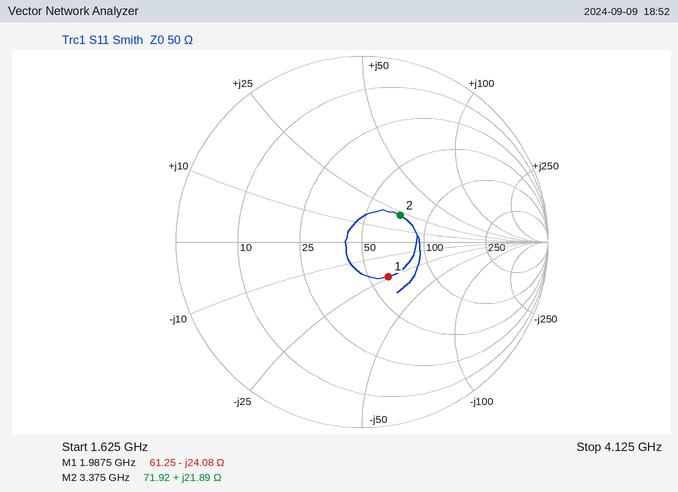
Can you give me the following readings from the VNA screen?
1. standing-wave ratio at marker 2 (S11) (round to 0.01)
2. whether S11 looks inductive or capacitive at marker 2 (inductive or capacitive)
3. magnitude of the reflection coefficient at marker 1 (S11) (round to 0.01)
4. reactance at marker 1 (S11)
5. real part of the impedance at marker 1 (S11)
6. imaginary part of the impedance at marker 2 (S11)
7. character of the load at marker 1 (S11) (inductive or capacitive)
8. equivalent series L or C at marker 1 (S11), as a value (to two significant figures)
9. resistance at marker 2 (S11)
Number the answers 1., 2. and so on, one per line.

1. 1.67
2. inductive
3. 0.23
4. -24.08 Ω
5. 61.25 Ω
6. +21.89 Ω
7. capacitive
8. 3.3 pF
9. 71.92 Ω
